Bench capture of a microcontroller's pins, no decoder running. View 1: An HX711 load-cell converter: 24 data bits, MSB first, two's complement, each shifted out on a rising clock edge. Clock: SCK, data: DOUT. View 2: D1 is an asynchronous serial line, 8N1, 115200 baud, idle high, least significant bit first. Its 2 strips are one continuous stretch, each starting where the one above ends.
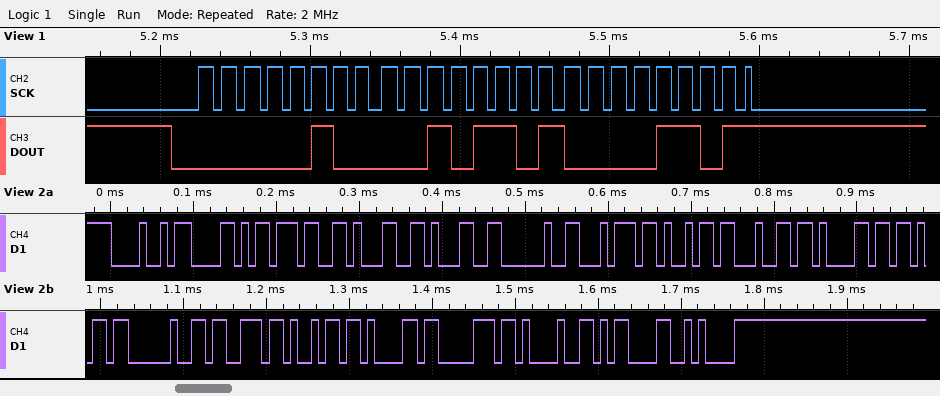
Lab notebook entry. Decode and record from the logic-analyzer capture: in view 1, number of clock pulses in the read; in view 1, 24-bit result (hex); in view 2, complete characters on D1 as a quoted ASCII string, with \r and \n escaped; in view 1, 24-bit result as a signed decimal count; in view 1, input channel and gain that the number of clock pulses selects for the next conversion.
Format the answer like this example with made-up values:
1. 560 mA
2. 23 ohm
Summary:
1. 25
2. 0x042D0D
3. "HX711 tidak siap!\r\n"
4. 273677
5. channel A, gain 128
